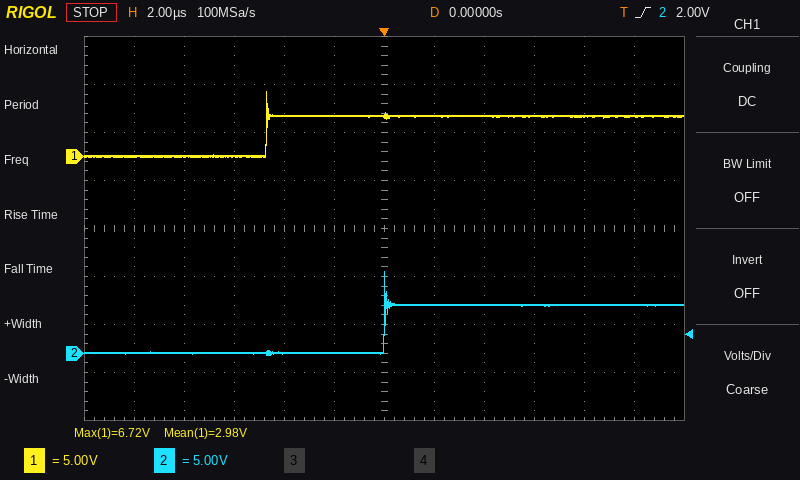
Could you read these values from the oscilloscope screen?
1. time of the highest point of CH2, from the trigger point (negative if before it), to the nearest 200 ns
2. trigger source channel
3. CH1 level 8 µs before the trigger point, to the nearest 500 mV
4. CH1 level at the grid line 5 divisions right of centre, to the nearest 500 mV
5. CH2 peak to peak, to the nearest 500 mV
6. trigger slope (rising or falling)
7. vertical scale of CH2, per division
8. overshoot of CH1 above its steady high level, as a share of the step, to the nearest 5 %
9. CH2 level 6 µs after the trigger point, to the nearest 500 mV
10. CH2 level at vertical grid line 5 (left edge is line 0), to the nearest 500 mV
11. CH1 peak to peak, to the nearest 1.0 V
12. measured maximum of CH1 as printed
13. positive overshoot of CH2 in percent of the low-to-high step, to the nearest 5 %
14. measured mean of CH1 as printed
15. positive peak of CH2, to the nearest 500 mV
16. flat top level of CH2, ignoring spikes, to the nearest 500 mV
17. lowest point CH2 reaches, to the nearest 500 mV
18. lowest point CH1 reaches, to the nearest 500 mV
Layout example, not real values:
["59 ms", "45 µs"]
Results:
["0.0 µs", "CH2", "0.0 V", "4.0 V", "8.5 V", "rising", "5 V", "60 %", "5.0 V", "0.0 V", "7.0 V", "6.72 V", "70 %", "2.98 V", "8.5 V", "5.0 V", "0.0 V", "0.0 V"]
